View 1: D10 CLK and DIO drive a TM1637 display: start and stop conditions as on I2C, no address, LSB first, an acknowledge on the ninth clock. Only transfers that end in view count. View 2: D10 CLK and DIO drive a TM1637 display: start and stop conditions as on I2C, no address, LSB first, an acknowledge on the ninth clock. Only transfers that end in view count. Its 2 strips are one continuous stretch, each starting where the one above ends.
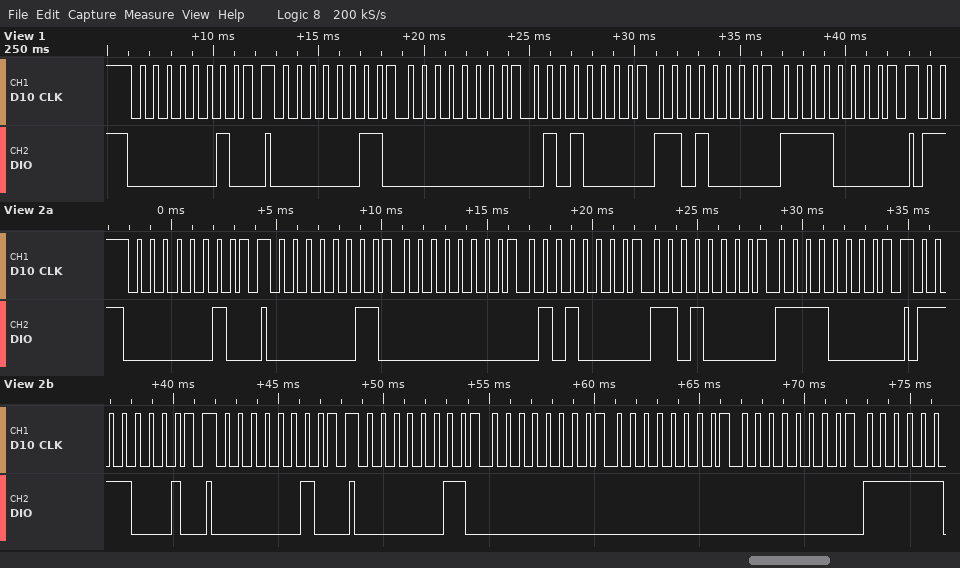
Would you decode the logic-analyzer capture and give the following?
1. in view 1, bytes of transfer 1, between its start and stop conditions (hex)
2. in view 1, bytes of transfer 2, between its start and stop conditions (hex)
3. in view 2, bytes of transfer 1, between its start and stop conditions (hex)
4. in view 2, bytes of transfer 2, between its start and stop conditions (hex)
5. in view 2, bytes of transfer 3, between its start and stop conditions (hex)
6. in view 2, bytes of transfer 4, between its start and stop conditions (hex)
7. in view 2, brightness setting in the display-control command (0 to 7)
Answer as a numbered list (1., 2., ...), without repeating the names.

1. 40
2. C0 00 0A 0B 0F
3. 40
4. C0 00 0A 0B 0F
5. 8F
6. 40
7. 7
